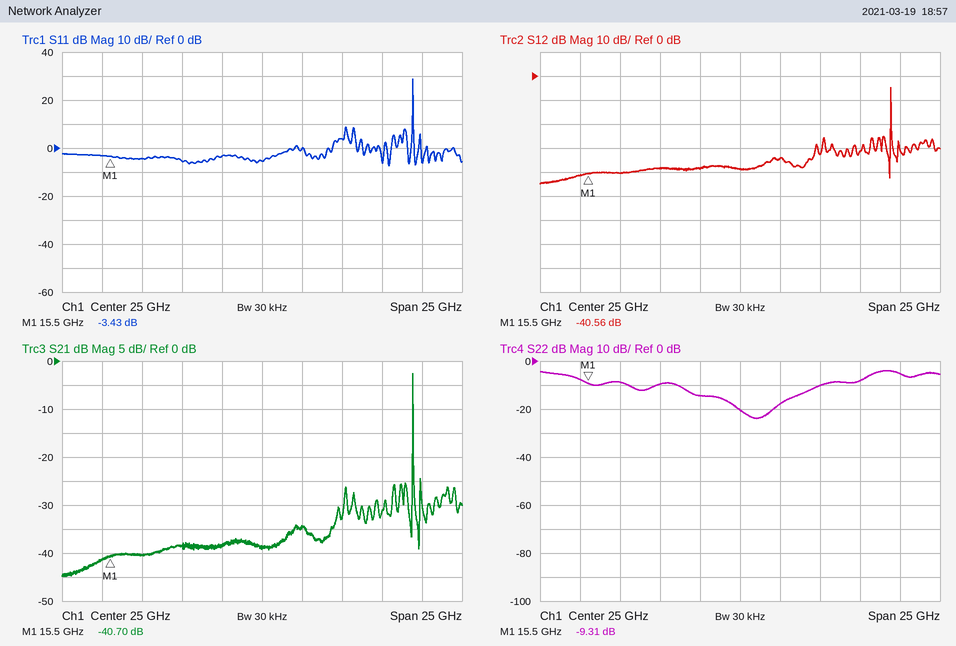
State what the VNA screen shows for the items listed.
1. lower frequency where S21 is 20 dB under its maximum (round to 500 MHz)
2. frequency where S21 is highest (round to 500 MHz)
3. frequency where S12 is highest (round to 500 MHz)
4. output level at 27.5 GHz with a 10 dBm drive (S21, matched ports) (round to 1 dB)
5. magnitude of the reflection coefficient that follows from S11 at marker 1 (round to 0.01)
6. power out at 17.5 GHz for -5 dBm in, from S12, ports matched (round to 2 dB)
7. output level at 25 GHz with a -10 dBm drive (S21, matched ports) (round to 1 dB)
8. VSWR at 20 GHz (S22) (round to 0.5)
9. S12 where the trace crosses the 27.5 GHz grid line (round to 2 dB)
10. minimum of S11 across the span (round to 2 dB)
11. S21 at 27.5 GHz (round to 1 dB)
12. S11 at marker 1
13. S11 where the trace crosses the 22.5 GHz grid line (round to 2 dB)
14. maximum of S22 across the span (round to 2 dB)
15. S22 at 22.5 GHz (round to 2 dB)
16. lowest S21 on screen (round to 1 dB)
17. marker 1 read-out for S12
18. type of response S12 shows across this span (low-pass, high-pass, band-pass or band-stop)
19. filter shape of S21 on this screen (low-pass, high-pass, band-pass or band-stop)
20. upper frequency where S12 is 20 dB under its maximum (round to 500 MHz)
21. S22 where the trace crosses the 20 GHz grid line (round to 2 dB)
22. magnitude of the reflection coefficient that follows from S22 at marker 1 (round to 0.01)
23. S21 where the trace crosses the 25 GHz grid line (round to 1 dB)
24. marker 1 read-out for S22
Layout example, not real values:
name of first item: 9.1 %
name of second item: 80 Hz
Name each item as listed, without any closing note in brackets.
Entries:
lower frequency where S21 is 20 dB under its maximum: 34.5 GHz
frequency where S21 is highest: 34.5 GHz
frequency where S12 is highest: 34.5 GHz
output level at 27.5 GHz with a 10 dBm drive (S21, matched ports): -25 dBm
magnitude of the reflection coefficient that follows from S11 at marker 1: 0.67
power out at 17.5 GHz for -5 dBm in, from S12, ports matched: -46 dBm
output level at 25 GHz with a -10 dBm drive (S21, matched ports): -49 dBm
VSWR at 20 GHz (S22): 2.0
S12 where the trace crosses the 27.5 GHz grid line: -34 dB
minimum of S11 across the span: -8 dB
S21 at 27.5 GHz: -35 dB
S11 at marker 1: -3.43 dB
S11 where the trace crosses the 22.5 GHz grid line: -4 dB
maximum of S22 across the span: -4 dB
S22 at 22.5 GHz: -14 dB
lowest S21 on screen: -45 dB
marker 1 read-out for S12: -40.56 dB
type of response S12 shows across this span: band-pass
filter shape of S21 on this screen: band-pass
upper frequency where S12 is 20 dB under its maximum: 34.5 GHz
S22 where the trace crosses the 20 GHz grid line: -10 dB
magnitude of the reflection coefficient that follows from S22 at marker 1: 0.34
S21 where the trace crosses the 25 GHz grid line: -39 dB
marker 1 read-out for S22: -9.31 dB
